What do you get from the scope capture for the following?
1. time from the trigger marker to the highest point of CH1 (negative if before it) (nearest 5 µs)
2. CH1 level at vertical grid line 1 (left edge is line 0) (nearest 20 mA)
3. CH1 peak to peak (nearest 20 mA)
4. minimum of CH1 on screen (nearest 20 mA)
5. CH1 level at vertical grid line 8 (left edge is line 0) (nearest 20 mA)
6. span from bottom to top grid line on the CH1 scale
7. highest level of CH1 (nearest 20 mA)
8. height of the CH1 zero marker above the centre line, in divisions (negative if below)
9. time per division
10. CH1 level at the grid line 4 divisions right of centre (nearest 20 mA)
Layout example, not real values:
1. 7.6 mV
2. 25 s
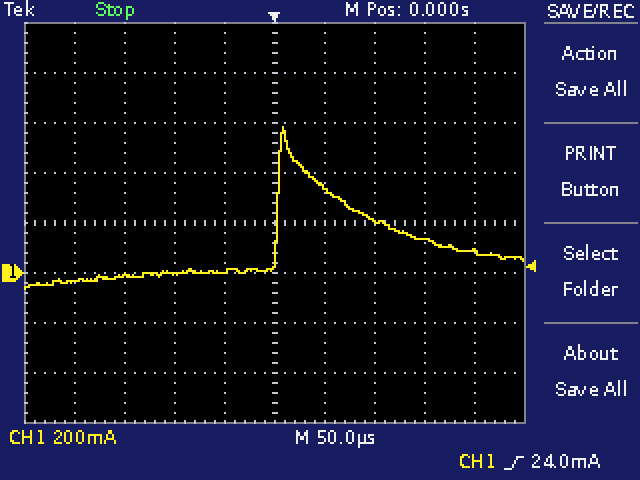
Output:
1. +10 µs
2. -40 mA
3. 640 mA
4. -60 mA
5. 140 mA
6. 1.6 A
7. 580 mA
8. -1.0 div
9. 50 µs
10. 80 mA
